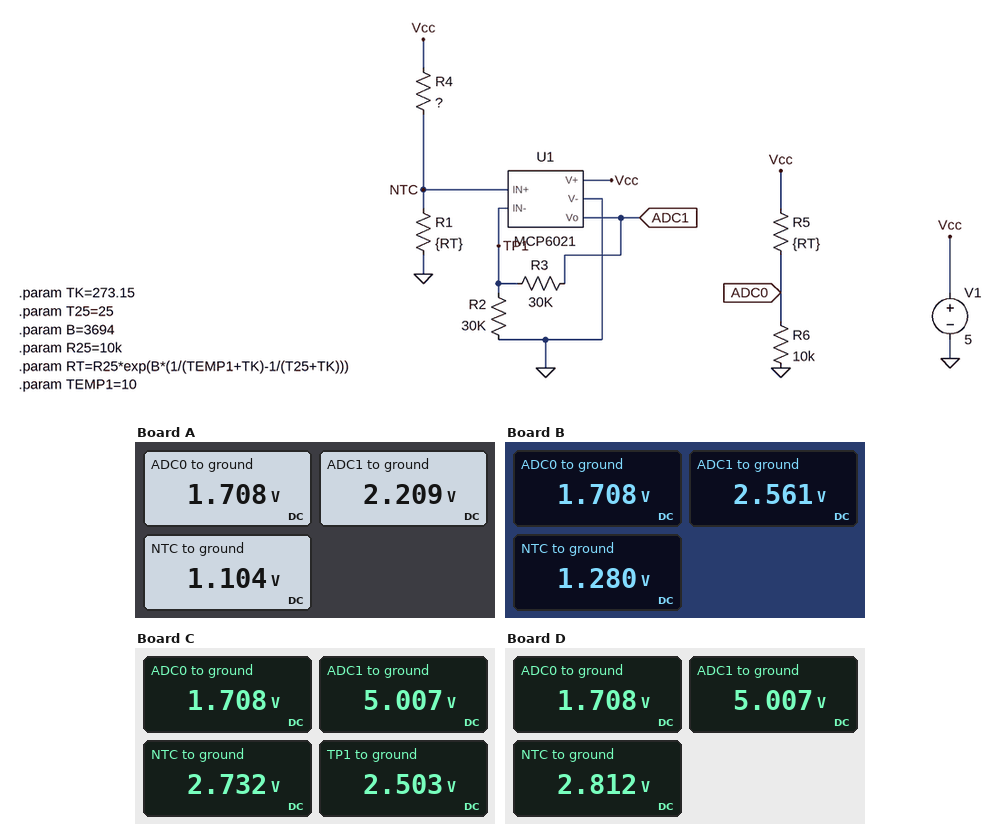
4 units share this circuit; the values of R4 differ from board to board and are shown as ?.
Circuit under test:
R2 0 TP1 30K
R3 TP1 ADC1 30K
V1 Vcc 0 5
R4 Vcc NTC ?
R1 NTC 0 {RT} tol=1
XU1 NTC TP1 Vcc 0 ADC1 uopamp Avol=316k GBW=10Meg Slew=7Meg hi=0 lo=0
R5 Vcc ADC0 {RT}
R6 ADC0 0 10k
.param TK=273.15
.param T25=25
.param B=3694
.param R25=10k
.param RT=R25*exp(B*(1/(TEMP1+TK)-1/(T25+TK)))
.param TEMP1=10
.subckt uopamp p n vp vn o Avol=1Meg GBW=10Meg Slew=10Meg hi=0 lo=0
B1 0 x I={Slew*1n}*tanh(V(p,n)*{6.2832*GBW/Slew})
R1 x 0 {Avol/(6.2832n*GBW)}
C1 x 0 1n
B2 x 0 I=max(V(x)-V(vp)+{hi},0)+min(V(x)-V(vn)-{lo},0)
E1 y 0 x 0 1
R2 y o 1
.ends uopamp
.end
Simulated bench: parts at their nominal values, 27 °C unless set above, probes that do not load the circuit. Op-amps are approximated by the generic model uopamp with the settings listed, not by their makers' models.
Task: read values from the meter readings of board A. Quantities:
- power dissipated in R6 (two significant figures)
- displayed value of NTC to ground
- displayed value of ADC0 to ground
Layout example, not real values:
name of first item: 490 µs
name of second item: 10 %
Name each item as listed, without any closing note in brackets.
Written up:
power dissipated in R6: 290 µW
displayed value of NTC to ground: 1.104 V
displayed value of ADC0 to ground: 1.708 V
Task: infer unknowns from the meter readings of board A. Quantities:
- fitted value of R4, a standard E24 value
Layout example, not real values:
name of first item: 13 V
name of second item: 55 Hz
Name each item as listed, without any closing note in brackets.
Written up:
fitted value of R4, a standard E24 value: 68 kΩ
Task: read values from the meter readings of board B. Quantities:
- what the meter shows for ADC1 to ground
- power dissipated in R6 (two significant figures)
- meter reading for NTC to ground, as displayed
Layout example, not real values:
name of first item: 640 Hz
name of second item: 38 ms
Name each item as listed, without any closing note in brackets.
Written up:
what the meter shows for ADC1 to ground: 2.561 V
power dissipated in R6: 290 µW
meter reading for NTC to ground, as displayed: 1.280 V
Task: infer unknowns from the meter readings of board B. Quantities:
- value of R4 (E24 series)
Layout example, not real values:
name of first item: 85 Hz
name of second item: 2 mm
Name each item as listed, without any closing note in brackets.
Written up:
value of R4: 56 kΩ
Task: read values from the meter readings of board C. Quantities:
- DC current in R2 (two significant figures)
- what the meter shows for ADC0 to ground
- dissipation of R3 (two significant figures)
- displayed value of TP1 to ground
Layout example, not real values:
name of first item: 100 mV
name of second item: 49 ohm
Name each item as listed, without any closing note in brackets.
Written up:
DC current in R2: 83 µA
what the meter shows for ADC0 to ground: 1.708 V
dissipation of R3: 210 µW
displayed value of TP1 to ground: 2.503 V
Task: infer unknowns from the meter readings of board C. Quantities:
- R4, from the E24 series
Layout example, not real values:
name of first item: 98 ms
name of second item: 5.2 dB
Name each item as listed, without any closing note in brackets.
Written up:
R4, from the E24 series: 16 kΩ
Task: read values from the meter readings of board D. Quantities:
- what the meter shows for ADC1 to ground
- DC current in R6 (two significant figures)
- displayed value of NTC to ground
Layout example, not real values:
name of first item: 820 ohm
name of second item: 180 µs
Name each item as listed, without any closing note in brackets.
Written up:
what the meter shows for ADC1 to ground: 5.007 V
DC current in R6: 170 µA
displayed value of NTC to ground: 2.812 V
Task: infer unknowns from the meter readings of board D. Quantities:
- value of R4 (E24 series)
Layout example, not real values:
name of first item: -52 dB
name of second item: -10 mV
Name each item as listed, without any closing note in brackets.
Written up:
value of R4: 15 kΩ
